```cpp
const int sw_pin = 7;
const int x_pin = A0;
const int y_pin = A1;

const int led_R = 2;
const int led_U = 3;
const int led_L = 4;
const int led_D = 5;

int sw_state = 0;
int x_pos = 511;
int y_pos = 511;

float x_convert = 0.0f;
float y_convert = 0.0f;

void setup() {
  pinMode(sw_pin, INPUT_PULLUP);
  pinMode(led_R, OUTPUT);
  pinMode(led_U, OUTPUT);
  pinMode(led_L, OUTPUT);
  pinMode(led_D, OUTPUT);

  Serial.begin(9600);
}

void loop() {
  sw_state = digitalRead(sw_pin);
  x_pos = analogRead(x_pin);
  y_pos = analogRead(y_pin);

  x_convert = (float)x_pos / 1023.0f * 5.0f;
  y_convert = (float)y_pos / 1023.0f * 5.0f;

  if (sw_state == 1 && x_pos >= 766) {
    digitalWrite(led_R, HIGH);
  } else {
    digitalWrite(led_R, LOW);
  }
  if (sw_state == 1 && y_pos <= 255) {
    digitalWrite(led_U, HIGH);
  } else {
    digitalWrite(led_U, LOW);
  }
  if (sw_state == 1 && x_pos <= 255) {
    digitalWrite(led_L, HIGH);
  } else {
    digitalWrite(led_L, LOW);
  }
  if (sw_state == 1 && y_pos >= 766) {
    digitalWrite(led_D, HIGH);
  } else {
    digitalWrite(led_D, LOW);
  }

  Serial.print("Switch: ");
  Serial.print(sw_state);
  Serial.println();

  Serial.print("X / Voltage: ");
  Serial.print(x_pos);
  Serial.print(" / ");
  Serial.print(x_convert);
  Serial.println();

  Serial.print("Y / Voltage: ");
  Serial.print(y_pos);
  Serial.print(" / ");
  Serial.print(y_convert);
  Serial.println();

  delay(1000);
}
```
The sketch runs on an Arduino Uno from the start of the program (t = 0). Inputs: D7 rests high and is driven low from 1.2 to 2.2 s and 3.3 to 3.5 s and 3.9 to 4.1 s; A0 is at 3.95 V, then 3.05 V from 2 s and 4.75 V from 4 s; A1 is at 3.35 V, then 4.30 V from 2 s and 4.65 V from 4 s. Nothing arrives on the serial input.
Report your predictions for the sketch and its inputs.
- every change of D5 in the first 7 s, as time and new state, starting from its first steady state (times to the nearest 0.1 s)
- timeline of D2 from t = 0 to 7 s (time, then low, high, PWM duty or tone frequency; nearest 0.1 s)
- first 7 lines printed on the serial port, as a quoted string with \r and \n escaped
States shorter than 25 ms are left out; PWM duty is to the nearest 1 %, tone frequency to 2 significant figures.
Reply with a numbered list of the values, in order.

1. 0 s low; 3 s high; 4 s low; 5 s high
2. 0 s high; 2 s low; 5 s high
3. "Switch: 1\r\nX / Voltage: 808 / 3.95\r\nY / Voltage: 686 / 3.35\r\nSwitch: 1\r\nX / Voltage: 808 / 3.95\r\nY / Voltage: 686 / 3.35\r\nSwitch: 0\r\n"
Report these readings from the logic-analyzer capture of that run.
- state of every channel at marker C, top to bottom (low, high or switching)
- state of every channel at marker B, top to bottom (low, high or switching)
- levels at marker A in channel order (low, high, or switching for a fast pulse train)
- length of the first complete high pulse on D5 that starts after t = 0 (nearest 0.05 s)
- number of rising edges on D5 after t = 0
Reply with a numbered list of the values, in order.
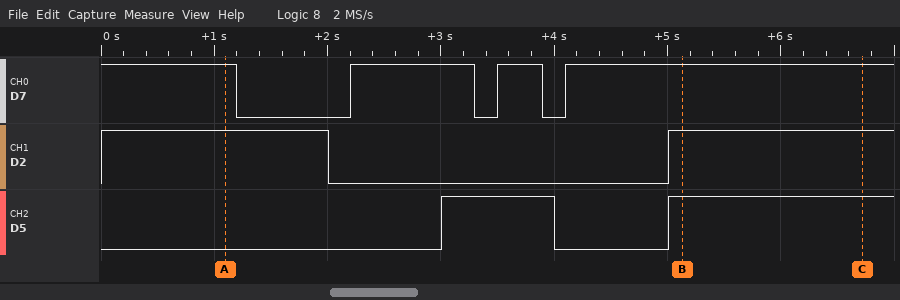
1. D7 high, D2 high, D5 high
2. D7 high, D2 high, D5 high
3. D7 high, D2 high, D5 low
4. 1.00 s
5. 2
